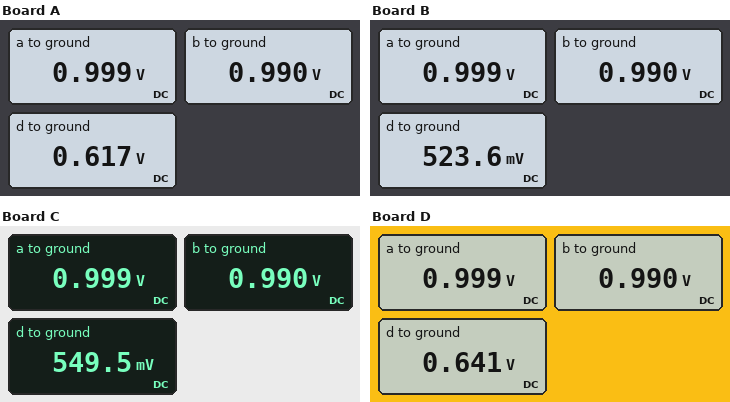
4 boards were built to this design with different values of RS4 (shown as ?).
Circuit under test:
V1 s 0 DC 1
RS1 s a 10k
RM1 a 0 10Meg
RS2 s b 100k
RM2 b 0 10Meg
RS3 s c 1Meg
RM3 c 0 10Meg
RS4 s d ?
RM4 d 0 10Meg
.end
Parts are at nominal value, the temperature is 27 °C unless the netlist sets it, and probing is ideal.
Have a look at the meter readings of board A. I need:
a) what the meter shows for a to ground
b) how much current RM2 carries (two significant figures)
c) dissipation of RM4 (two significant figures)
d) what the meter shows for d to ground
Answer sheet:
0.999 V
99 nA
38 nW
0.617 V
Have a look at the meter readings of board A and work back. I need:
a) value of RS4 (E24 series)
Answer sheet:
6.2 MΩ
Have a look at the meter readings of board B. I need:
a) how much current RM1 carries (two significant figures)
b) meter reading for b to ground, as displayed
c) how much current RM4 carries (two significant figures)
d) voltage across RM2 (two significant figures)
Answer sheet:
100 nA
0.990 V
52 nA
990 mV
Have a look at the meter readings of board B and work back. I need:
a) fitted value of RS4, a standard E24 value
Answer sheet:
9.1 MΩ
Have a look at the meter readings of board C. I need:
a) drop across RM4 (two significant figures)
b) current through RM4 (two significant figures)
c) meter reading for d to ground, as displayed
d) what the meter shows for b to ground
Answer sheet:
550 mV
55 nA
549.5 mV
0.990 V
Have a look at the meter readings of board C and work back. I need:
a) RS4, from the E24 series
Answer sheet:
8.2 MΩ
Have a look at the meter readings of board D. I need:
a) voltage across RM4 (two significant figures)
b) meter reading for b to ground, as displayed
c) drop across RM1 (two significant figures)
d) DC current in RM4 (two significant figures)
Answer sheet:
640 mV
0.990 V
1.0 V
64 nA
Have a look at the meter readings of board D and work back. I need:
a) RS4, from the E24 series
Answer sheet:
5.6 MΩ
